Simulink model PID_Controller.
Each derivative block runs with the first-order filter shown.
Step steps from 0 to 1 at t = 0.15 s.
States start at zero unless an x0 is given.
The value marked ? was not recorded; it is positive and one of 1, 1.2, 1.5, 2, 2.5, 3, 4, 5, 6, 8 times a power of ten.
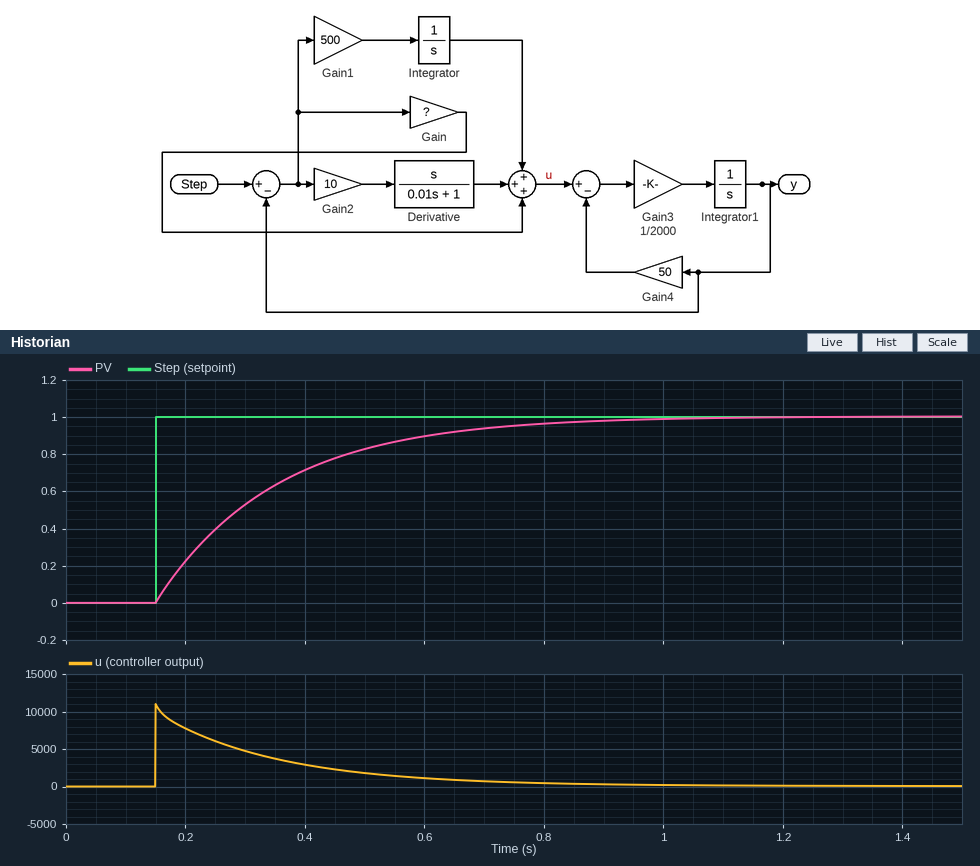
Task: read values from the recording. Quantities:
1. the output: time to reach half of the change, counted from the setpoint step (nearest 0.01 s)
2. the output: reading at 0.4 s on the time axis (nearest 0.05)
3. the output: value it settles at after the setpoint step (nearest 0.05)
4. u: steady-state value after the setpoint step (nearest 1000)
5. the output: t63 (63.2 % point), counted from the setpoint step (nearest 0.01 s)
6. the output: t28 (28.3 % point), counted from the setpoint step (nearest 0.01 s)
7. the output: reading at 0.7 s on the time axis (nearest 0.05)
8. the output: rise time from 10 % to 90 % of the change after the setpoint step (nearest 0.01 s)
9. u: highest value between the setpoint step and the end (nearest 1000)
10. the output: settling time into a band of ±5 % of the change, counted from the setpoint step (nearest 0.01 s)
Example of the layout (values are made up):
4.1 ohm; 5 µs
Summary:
0.14 s; 0.70; 1.00; 0; 0.20 s; 0.07 s; 0.95; 0.44 s; 11000; 0.60 s
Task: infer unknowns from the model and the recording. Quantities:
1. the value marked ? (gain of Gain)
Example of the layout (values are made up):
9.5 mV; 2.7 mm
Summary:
10000
